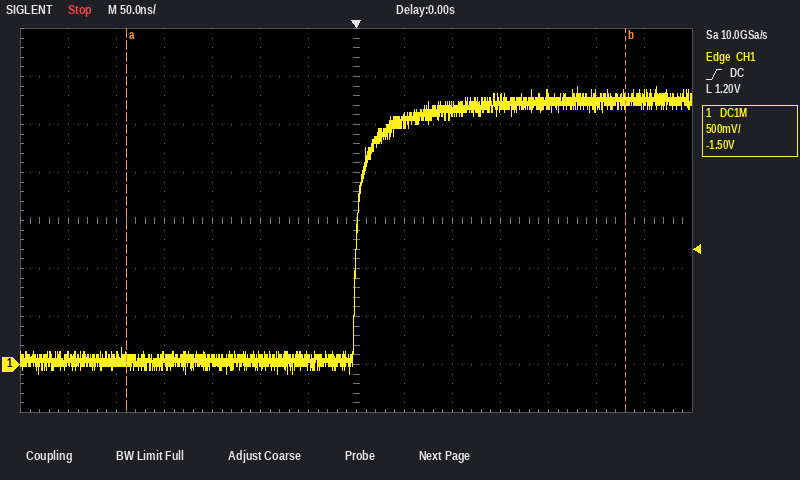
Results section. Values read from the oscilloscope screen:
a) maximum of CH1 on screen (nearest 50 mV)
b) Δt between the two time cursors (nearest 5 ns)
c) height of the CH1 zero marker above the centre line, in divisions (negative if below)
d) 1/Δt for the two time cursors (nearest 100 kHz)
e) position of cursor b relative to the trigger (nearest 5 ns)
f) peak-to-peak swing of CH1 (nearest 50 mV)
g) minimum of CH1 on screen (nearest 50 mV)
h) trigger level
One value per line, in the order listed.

2.90 V
520 ns
-3.0 div
1.9 MHz
+280 ns
3.00 V
-100 mV
1.20 V
